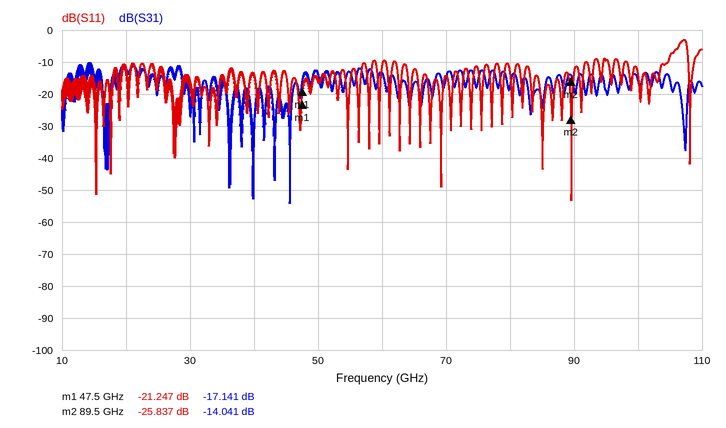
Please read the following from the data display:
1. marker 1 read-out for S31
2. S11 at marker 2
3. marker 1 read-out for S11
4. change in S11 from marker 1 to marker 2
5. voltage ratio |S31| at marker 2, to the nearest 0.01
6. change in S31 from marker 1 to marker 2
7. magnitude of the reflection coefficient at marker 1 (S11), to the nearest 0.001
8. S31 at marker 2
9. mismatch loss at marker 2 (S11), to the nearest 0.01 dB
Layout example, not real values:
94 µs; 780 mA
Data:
-17.141 dB; -25.837 dB; -21.247 dB; -4.590 dB; 0.20; 3.100 dB; 0.087; -14.041 dB; 0.01 dB
